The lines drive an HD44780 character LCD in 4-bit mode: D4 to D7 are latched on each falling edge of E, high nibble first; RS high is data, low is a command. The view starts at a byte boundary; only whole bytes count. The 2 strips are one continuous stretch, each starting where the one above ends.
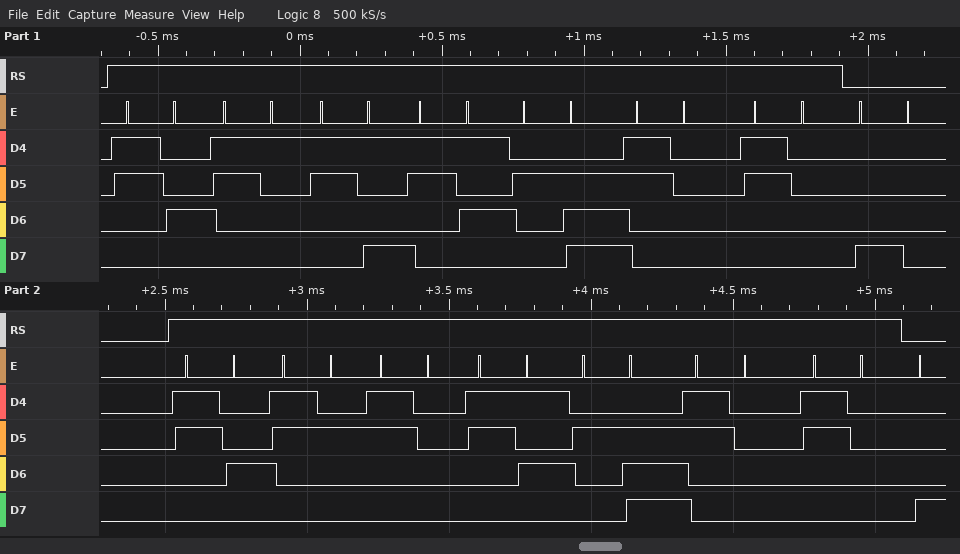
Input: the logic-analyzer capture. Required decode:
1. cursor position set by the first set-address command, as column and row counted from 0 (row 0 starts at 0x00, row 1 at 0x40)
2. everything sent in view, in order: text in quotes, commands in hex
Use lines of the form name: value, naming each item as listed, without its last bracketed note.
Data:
cursor position set by the first set-address command, as column and row counted from 0: column 0, row 0
everything sent in view, in order: text in quotes, commands in hex: "4195.00" 0x80 "4205.00"
